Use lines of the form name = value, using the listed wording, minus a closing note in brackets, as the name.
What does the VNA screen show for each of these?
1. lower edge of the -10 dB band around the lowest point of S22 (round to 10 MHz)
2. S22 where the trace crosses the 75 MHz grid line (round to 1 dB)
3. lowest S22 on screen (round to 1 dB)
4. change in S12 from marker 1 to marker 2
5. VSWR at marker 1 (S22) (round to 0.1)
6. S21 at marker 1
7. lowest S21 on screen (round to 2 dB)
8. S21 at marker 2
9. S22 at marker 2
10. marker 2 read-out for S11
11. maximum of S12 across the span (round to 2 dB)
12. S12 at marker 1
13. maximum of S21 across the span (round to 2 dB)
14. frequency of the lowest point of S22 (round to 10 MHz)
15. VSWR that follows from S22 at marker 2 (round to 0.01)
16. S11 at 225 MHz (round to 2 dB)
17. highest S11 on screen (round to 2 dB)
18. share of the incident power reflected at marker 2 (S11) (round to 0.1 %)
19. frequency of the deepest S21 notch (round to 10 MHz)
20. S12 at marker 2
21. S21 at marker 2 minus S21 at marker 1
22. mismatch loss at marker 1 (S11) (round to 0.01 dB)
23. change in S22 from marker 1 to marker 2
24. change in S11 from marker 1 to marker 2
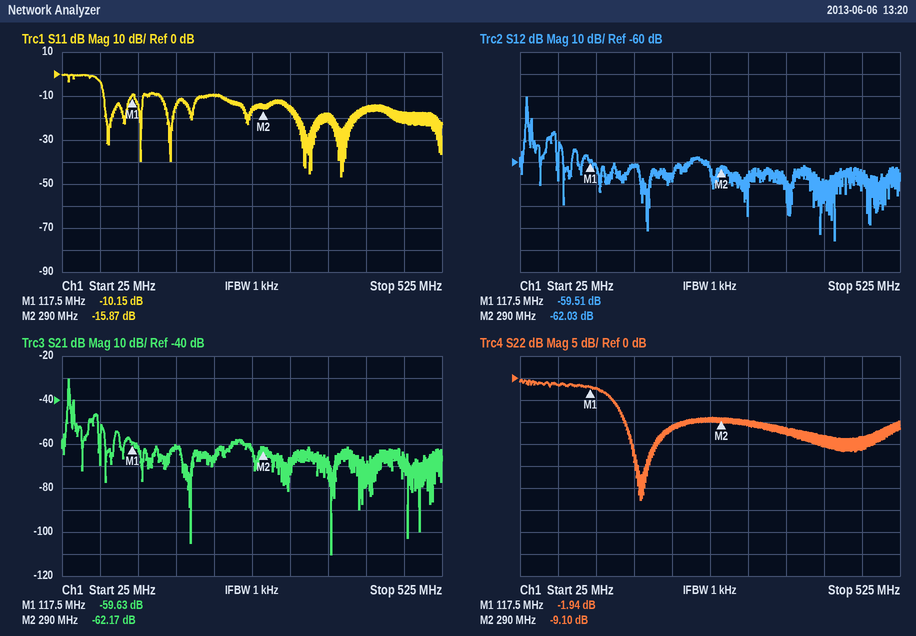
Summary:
lower edge of the -10 dB band around the lowest point of S22 = 160 MHz
S22 where the trace crosses the 75 MHz grid line = -2 dB
lowest S22 on screen = -28 dB
change in S12 from marker 1 to marker 2 = -2.52 dB
VSWR at marker 1 (S22) = 9.0
S21 at marker 1 = -59.63 dB
lowest S21 on screen = -110 dB
S21 at marker 2 = -62.17 dB
S22 at marker 2 = -9.10 dB
marker 2 read-out for S11 = -15.87 dB
maximum of S12 across the span = -30 dB
S12 at marker 1 = -59.51 dB
maximum of S21 across the span = -30 dB
frequency of the lowest point of S22 = 180 MHz
VSWR that follows from S22 at marker 2 = 2.08
S11 at 225 MHz = -10 dB
highest S11 on screen = 0 dB
share of the incident power reflected at marker 2 (S11) = 2.6 %
frequency of the deepest S21 notch = 380 MHz
S12 at marker 2 = -62.03 dB
S21 at marker 2 minus S21 at marker 1 = -2.54 dB
mismatch loss at marker 1 (S11) = 0.44 dB
change in S22 from marker 1 to marker 2 = -7.16 dB
change in S11 from marker 1 to marker 2 = -5.72 dB
